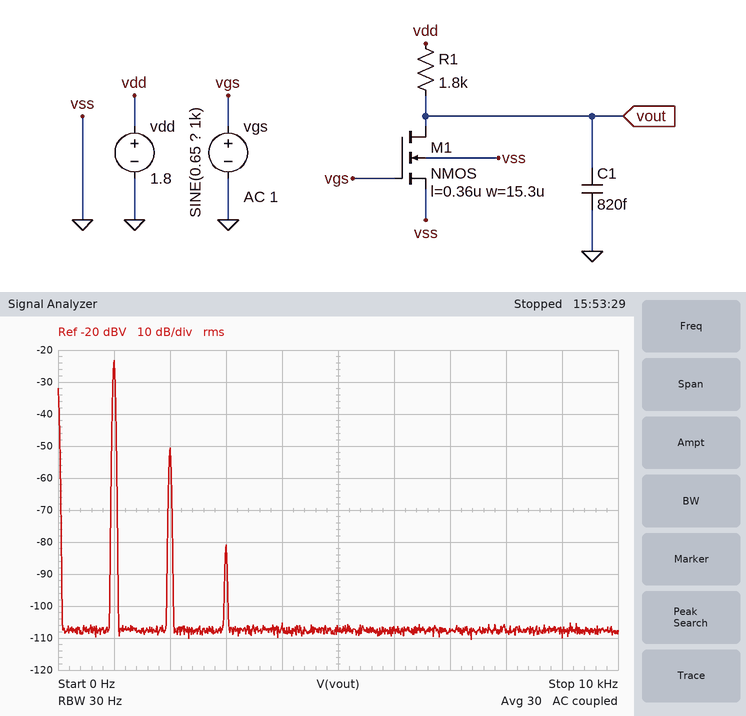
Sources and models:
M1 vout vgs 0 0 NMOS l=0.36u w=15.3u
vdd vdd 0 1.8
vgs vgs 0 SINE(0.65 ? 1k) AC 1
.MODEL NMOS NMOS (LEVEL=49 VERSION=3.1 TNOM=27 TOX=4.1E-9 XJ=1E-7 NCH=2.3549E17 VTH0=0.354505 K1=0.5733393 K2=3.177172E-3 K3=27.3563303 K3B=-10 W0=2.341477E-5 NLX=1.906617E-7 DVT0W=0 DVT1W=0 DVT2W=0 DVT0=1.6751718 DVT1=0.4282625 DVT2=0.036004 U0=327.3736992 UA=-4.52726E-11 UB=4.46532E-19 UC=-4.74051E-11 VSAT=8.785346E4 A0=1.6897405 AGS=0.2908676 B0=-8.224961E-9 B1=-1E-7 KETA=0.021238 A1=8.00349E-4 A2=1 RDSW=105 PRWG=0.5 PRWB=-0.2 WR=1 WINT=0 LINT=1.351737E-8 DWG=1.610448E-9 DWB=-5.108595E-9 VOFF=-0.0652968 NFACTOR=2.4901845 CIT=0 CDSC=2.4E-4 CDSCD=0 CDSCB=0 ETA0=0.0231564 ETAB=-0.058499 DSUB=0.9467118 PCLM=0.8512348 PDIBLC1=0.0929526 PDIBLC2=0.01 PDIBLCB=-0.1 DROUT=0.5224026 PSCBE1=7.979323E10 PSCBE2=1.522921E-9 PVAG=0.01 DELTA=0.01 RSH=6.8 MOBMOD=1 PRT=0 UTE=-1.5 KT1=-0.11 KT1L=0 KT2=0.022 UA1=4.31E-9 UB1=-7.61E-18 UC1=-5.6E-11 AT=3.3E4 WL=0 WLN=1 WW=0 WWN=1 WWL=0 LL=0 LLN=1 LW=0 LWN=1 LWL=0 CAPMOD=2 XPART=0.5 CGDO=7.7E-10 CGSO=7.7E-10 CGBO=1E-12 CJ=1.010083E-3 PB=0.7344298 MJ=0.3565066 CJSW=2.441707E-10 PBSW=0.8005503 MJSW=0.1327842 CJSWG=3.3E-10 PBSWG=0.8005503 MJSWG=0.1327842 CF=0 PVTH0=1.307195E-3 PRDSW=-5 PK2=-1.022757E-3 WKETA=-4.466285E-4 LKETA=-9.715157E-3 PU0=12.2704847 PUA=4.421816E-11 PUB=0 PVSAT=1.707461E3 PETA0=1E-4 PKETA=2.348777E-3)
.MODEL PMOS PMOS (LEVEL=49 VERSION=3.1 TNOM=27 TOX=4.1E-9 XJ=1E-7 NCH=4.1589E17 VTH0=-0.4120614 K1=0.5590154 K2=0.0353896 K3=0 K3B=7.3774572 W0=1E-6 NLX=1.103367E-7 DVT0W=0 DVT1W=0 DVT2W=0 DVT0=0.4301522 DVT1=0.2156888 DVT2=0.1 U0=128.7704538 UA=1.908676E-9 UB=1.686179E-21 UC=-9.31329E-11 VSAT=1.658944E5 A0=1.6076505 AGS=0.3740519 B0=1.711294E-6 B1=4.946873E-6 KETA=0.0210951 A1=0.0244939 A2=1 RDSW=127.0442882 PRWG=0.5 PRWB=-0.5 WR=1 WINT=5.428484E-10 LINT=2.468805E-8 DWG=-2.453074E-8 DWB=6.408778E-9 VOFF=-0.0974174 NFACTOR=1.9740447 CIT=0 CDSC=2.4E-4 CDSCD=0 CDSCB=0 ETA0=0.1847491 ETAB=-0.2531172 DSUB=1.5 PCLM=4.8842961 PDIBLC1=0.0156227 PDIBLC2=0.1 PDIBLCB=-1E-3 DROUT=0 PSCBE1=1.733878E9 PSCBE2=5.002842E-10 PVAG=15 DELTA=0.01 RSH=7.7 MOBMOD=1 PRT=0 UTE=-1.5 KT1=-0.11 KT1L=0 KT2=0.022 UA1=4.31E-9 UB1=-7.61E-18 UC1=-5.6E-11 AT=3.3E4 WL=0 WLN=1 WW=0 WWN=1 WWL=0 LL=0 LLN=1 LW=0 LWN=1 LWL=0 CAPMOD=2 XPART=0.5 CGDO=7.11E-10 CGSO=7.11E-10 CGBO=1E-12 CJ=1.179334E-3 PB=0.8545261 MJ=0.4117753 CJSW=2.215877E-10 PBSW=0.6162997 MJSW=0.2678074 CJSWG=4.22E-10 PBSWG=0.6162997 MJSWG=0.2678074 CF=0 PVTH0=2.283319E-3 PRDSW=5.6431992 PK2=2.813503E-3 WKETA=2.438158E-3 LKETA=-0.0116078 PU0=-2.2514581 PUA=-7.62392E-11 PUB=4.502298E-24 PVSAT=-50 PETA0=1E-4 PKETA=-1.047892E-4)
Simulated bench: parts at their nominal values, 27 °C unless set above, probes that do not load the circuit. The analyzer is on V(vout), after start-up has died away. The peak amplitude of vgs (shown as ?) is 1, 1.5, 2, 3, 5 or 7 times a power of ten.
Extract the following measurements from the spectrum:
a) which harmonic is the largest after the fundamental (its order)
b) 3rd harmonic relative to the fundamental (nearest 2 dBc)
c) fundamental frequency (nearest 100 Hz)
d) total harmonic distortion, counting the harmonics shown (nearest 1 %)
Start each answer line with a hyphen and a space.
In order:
- 2
- -58 dBc
- 1.0 kHz
- 4 %
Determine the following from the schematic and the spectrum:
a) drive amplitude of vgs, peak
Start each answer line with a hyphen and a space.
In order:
- 30 mV
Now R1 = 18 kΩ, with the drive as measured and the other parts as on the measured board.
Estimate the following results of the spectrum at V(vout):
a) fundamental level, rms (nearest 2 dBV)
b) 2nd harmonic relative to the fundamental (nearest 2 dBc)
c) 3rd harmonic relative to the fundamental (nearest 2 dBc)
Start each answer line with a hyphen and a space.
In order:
- -28 dBV
- -8 dBc
- -14 dBc
